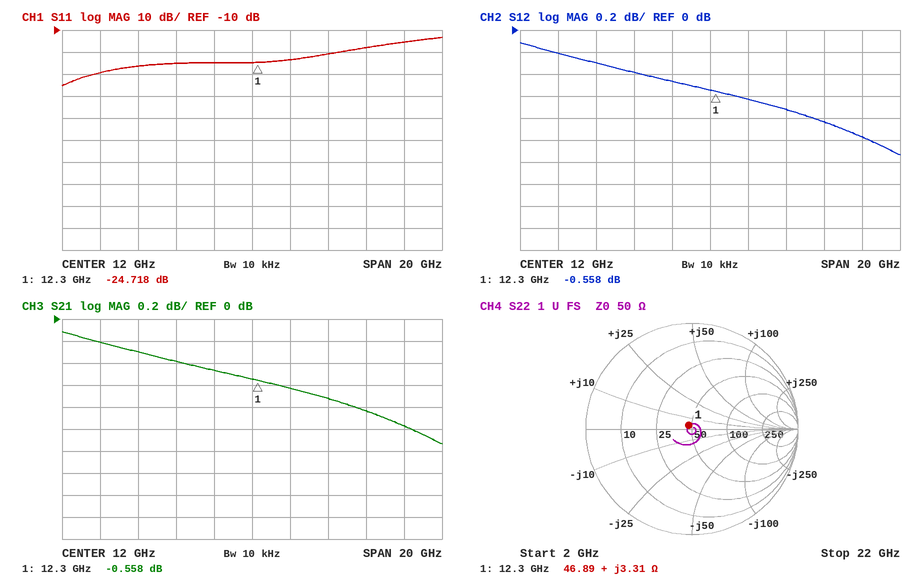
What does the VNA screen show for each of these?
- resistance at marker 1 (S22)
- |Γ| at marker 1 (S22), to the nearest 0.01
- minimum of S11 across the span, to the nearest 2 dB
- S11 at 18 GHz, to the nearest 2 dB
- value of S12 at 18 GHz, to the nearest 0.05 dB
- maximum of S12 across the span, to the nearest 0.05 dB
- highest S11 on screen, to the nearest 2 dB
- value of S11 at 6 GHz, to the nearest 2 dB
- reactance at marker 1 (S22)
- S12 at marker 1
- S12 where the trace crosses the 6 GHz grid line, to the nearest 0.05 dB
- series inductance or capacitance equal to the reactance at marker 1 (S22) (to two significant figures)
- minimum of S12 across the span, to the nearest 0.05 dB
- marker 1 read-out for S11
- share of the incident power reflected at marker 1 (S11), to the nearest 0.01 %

46.89 Ω
0.05
-36 dB
-18 dB
-0.85 dB
-0.10 dB
-14 dB
-26 dB
+3.31 Ω
-0.558 dB
-0.30 dB
43 pH
-1.15 dB
-24.718 dB
0.34 %
